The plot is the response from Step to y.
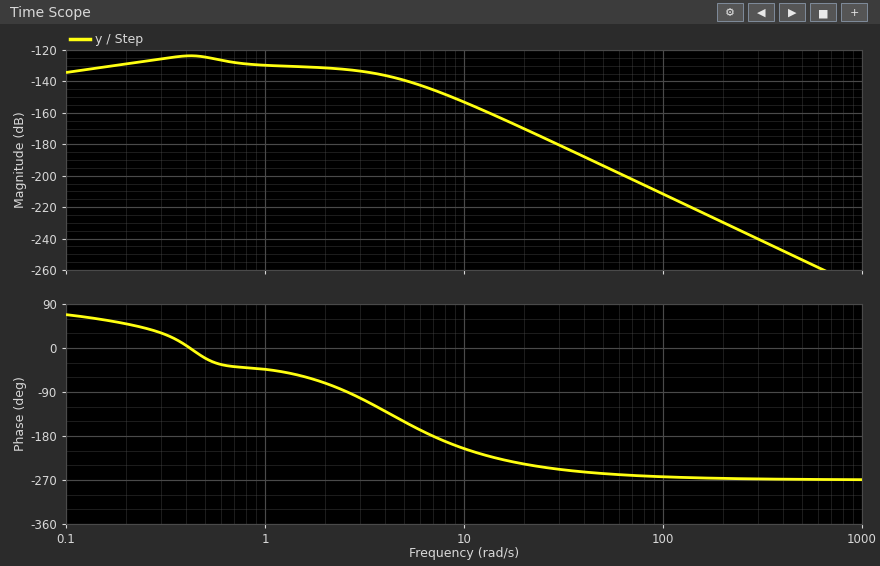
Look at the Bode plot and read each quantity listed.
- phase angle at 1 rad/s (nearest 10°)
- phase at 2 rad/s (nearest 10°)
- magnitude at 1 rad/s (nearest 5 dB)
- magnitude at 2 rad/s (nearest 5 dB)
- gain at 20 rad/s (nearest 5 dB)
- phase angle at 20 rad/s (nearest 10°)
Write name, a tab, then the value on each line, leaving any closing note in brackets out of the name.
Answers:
phase angle at 1 rad/s	-40°
phase at 2 rad/s	-70°
magnitude at 1 rad/s	-130 dB
magnitude at 2 rad/s	-130 dB
gain at 20 rad/s	-170 dB
phase angle at 20 rad/s	-240°
